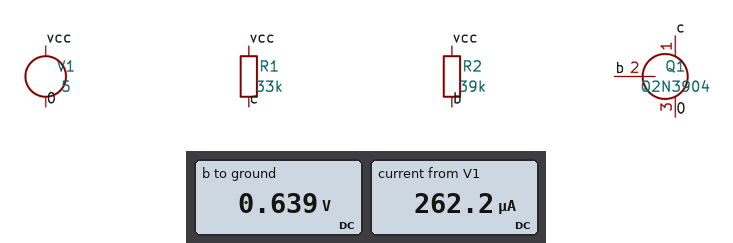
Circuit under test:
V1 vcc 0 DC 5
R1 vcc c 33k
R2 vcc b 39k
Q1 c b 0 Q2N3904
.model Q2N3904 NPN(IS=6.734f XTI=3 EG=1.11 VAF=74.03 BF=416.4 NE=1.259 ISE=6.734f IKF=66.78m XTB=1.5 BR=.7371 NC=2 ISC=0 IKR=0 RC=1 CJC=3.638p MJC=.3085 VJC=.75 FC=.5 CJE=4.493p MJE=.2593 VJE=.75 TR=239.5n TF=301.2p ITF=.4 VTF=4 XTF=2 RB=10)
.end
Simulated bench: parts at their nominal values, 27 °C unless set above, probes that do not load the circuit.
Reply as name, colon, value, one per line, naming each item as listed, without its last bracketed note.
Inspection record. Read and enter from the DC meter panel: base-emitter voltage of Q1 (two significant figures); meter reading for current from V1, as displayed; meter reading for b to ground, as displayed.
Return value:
base-emitter voltage of Q1: 640 mV
meter reading for current from V1, as displayed: 262.2 µA
meter reading for b to ground, as displayed: 0.639 V
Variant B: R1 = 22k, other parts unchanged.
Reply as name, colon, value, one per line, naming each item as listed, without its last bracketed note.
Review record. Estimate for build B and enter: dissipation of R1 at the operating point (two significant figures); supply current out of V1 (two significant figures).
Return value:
dissipation of R1 at the operating point: 1.1 mW
supply current out of V1: 340 µA
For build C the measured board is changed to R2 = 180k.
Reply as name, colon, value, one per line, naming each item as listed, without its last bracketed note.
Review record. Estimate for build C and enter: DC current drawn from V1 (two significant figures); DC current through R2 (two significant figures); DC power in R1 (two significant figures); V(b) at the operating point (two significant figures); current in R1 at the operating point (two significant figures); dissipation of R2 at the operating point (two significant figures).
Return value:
DC current drawn from V1: 170 µA
DC current through R2: 24 µA
DC power in R1: 740 µW
V(b) at the operating point: 620 mV
current in R1 at the operating point: 150 µA
dissipation of R2 at the operating point: 110 µW
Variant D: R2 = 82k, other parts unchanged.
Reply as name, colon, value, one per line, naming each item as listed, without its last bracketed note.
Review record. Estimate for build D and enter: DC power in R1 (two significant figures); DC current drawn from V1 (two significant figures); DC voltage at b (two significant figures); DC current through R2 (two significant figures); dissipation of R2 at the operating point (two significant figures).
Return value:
DC power in R1: 740 µW
DC current drawn from V1: 200 µA
DC voltage at b: 630 mV
DC current through R2: 53 µA
dissipation of R2 at the operating point: 230 µW
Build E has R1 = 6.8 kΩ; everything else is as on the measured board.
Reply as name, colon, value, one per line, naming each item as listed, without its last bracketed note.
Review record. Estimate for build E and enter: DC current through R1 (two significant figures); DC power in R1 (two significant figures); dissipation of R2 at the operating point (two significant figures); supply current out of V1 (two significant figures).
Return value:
DC current through R1: 730 µA
DC power in R1: 3.6 mW
dissipation of R2 at the operating point: 480 µW
supply current out of V1: 840 µA
